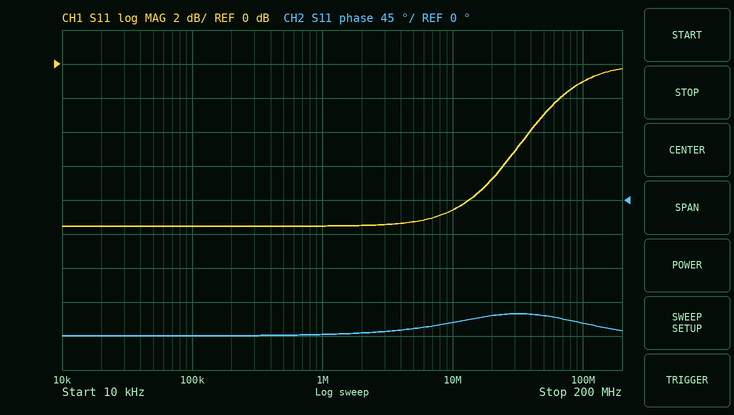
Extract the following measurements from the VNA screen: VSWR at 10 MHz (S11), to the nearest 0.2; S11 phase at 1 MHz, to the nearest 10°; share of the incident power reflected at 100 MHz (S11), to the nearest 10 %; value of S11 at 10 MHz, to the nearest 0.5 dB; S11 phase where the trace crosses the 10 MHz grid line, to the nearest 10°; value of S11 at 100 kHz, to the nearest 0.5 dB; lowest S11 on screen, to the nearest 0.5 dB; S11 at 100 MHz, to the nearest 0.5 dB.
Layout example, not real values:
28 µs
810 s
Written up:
2.2
-180°
80 %
-8.5 dB
-160°
-9.5 dB
-9.5 dB
-1.0 dB
